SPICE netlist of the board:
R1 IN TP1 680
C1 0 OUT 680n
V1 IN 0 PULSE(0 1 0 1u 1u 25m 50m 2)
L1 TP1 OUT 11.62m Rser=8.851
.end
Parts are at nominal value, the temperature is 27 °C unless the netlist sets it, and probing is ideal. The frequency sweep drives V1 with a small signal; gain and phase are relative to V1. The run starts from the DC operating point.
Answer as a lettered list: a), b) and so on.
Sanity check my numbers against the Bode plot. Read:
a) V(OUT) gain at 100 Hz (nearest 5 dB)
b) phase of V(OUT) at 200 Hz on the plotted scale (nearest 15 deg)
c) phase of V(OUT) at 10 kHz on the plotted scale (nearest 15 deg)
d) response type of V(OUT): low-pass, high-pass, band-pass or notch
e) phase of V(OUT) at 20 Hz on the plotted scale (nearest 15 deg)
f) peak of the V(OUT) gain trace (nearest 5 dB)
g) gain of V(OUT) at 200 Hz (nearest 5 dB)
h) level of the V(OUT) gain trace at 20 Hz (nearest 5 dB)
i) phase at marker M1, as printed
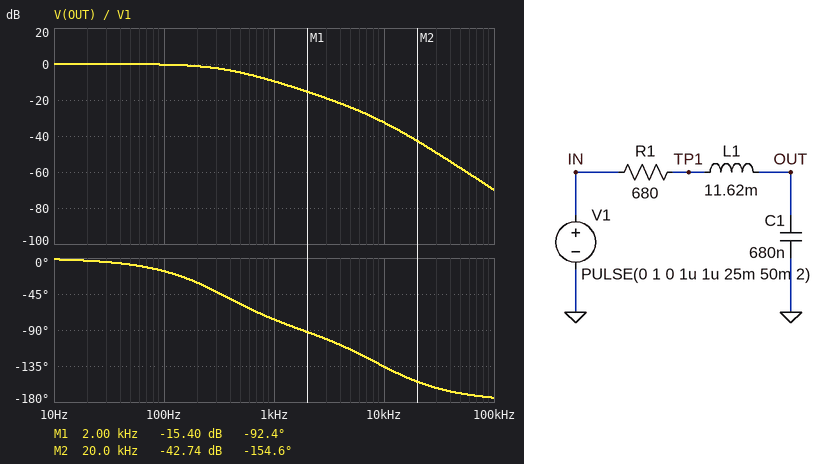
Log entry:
a) 0 dB
b) -30 deg
c) -135 deg
d) low-pass
e) 0 deg
f) 0 dB
g) 0 dB
h) 0 dB
i) -92.4 deg
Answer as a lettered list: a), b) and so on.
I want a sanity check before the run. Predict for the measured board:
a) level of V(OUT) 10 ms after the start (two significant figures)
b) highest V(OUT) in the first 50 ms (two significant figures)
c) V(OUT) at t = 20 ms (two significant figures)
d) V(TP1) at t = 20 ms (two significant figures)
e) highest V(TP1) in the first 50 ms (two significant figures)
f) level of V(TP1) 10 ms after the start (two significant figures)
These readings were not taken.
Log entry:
a) 1.0 V
b) 1.0 V
c) 1.0 V
d) 1.0 V
e) 1.0 V
f) 1.0 V
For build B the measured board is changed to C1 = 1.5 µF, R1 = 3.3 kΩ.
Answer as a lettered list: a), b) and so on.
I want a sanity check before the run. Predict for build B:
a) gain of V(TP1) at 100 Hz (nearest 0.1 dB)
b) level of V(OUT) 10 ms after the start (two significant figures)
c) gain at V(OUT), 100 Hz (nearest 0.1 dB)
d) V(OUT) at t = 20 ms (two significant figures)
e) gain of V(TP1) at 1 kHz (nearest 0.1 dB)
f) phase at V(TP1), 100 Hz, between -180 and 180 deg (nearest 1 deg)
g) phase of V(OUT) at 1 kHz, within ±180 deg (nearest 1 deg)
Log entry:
a) -10.4 dB
b) 870 mV
c) -10.3 dB
d) 980 mV
e) -39.7 dB
f) -72 deg
g) -89 deg
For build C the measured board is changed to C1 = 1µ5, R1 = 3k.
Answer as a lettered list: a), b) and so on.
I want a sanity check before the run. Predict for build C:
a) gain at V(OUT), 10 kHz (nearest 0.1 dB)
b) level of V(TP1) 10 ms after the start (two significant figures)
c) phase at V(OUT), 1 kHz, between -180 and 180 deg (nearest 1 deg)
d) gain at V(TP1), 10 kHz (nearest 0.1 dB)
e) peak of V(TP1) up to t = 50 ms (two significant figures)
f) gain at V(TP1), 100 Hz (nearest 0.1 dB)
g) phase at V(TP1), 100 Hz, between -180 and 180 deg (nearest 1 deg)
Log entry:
a) -49.3 dB
b) 890 mV
c) -89 deg
d) -12.7 dB
e) 1.0 V
f) -9.6 dB
g) -70 deg
